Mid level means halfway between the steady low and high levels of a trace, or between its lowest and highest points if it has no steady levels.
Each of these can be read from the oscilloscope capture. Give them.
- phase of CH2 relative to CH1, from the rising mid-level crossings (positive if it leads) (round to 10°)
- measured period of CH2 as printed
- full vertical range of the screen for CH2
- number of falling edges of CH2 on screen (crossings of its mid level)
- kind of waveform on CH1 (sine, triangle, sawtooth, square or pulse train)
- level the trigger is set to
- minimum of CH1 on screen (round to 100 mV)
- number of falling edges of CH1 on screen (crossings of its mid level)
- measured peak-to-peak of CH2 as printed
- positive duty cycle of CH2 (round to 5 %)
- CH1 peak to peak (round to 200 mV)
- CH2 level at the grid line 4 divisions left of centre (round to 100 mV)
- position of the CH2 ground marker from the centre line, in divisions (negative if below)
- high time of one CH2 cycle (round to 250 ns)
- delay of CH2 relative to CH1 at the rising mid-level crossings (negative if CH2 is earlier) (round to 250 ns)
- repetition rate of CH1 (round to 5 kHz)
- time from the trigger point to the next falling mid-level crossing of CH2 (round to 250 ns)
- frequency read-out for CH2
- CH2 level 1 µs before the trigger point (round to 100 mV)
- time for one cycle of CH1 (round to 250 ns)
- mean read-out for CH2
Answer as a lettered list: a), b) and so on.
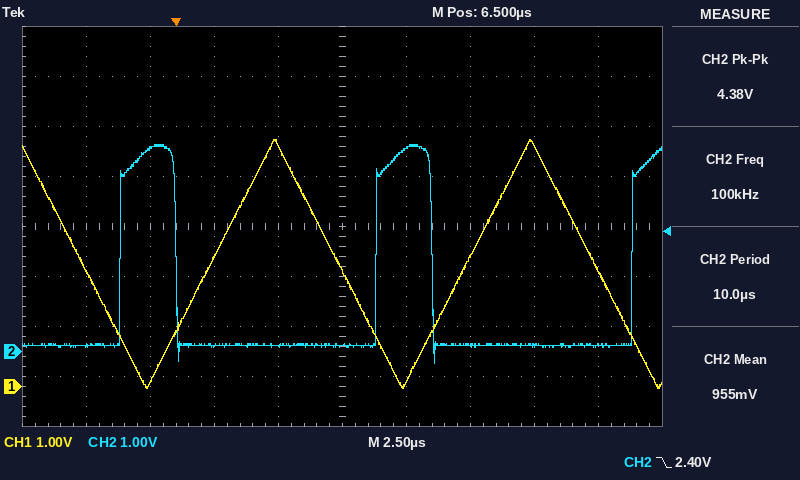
a) +130°
b) 10.0 µs
c) 8 V
d) 2
e) triangle
f) 2.40 V
g) 0.0 V
h) 3
i) 4.38 V
j) 20 %
k) 5.0 V
l) 100 mV
m) -2.5 div
n) 2.25 µs
o) -3.50 µs
p) 100 kHz
q) 10.00 µs
r) 100 kHz
s) 4.1 V
t) 10.00 µs
u) 955 mV
